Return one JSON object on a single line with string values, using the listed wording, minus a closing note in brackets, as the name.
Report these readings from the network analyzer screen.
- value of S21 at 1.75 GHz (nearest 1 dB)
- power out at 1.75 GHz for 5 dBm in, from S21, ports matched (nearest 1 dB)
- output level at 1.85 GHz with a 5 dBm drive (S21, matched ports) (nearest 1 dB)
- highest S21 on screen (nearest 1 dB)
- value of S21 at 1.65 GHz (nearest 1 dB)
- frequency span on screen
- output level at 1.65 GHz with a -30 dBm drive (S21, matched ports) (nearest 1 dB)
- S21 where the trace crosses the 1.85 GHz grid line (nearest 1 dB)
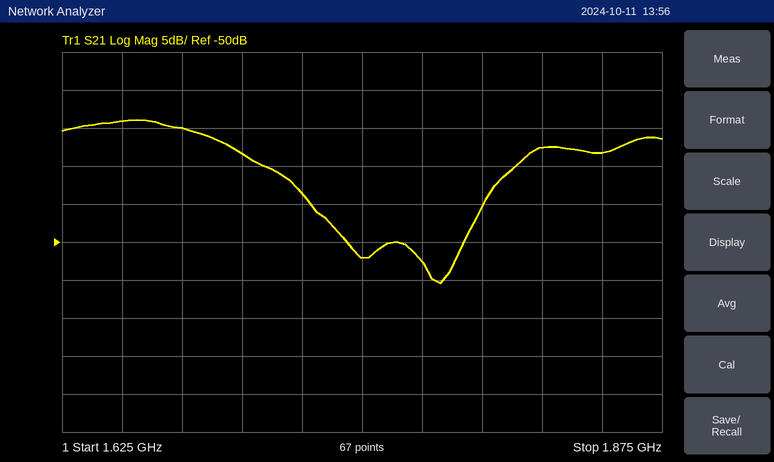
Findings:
{"value of S21 at 1.75 GHz": "-52 dB", "power out at 1.75 GHz for 5 dBm in, from S21, ports matched": "-47 dBm", "output level at 1.85 GHz with a 5 dBm drive (S21, matched ports)": "-33 dBm", "highest S21 on screen": "-34 dB", "value of S21 at 1.65 GHz": "-34 dB", "frequency span on screen": "250 MHz", "output level at 1.65 GHz with a -30 dBm drive (S21, matched ports)": "-64 dBm", "S21 where the trace crosses the 1.85 GHz grid line": "-38 dB"}
